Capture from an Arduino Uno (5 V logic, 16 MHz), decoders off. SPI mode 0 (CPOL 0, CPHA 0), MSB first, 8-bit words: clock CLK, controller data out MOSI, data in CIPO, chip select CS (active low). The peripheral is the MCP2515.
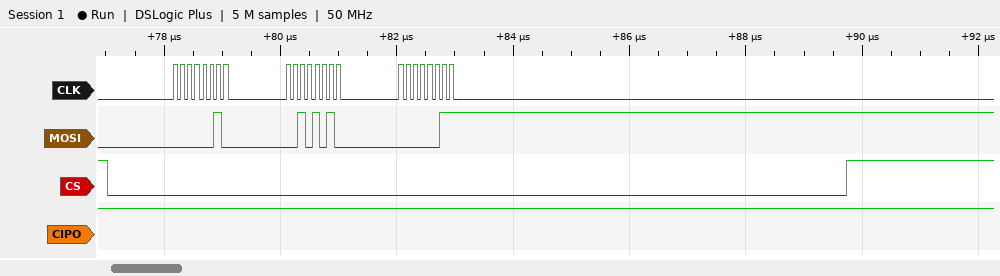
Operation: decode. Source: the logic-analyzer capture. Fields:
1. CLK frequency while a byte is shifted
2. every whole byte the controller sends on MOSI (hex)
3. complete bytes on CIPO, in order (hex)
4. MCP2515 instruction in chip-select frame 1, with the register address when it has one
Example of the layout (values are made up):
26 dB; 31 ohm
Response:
8 MHz; 02 2A 03; FF FF FF; WRITE 0x2A
